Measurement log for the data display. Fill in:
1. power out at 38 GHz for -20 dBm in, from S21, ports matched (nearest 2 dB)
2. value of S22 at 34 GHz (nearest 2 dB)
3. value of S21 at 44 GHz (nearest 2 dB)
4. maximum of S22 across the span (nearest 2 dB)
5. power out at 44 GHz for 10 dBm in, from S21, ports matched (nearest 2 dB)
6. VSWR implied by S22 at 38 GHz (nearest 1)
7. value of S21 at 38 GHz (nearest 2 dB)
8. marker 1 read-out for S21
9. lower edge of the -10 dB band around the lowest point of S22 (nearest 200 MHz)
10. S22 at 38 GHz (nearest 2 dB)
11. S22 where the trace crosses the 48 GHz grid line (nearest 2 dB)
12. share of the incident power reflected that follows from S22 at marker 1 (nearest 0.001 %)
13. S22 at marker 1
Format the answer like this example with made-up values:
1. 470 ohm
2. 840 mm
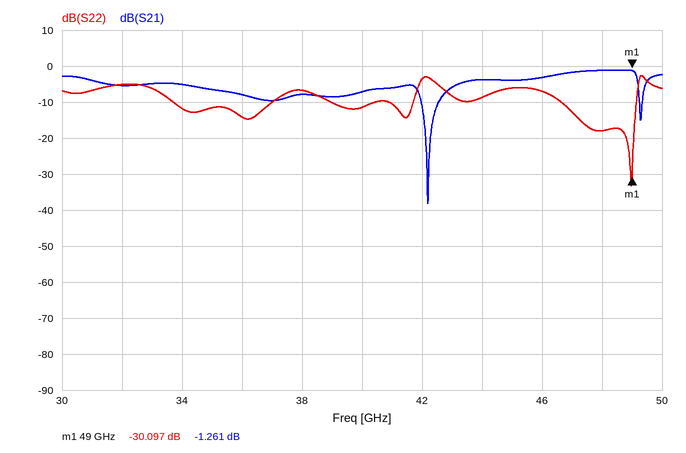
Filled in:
1. -28 dBm
2. -12 dB
3. -4 dB
4. -2 dB
5. 6 dBm
6. 3
7. -8 dB
8. -1.261 dB
9. 46.6 GHz
10. -6 dB
11. -18 dB
12. 0.098 %
13. -30.097 dB
